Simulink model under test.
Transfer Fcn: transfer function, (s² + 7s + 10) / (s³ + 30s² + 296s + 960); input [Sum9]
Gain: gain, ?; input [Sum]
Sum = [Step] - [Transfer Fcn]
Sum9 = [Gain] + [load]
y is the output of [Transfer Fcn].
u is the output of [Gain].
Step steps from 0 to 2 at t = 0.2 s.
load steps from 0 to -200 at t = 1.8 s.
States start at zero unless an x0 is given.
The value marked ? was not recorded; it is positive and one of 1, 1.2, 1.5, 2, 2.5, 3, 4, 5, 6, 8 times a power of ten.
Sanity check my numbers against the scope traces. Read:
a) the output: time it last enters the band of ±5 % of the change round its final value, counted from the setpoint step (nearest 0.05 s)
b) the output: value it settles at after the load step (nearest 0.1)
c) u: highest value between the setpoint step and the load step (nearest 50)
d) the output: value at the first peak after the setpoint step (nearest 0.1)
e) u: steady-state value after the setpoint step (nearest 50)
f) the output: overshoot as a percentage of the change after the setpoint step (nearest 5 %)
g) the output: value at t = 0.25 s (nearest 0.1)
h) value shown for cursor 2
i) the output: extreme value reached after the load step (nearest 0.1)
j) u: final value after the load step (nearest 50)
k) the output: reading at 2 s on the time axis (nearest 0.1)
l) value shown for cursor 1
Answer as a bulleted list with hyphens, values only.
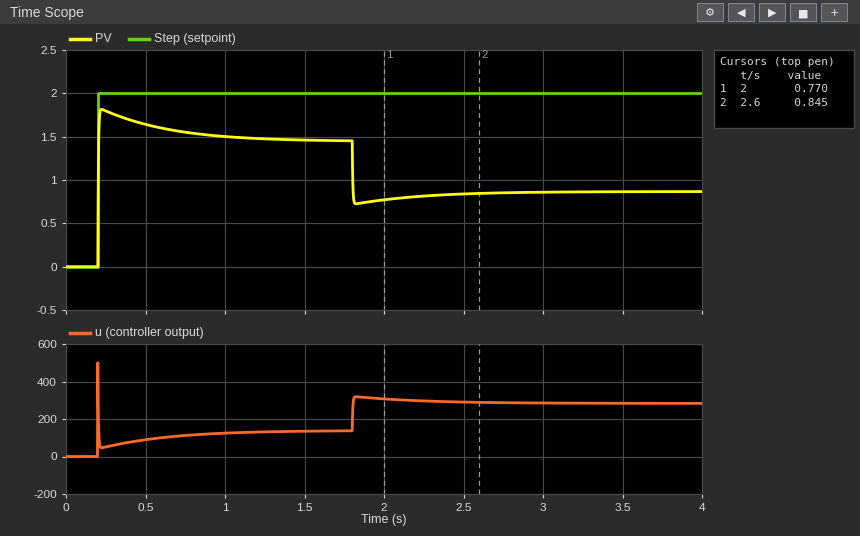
- 0.70 s
- 0.9
- 500
- 1.8
- 150
- 25 %
- 1.8
- 0.845
- 0.7
- 300
- 0.8
- 0.770
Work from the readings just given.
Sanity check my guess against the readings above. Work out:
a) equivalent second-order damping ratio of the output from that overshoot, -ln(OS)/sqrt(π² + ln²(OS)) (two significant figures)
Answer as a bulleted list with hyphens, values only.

- 0.40
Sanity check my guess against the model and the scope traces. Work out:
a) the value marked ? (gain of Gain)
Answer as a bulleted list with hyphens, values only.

- 250
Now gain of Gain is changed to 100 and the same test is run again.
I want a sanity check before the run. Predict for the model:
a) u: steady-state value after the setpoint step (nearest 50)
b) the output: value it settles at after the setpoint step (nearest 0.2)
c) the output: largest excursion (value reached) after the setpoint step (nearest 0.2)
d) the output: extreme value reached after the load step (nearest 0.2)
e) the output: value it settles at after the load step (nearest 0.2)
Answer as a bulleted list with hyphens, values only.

- 100
- 1.0
- 1.6
- -0.6
- 0.0
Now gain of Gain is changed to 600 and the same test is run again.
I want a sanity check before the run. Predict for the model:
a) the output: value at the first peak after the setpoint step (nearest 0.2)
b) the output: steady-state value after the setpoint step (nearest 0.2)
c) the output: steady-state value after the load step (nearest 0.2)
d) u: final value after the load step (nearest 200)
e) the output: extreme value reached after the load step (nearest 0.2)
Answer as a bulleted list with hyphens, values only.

- 2.0
- 1.8
- 1.4
- 400
- 1.4
